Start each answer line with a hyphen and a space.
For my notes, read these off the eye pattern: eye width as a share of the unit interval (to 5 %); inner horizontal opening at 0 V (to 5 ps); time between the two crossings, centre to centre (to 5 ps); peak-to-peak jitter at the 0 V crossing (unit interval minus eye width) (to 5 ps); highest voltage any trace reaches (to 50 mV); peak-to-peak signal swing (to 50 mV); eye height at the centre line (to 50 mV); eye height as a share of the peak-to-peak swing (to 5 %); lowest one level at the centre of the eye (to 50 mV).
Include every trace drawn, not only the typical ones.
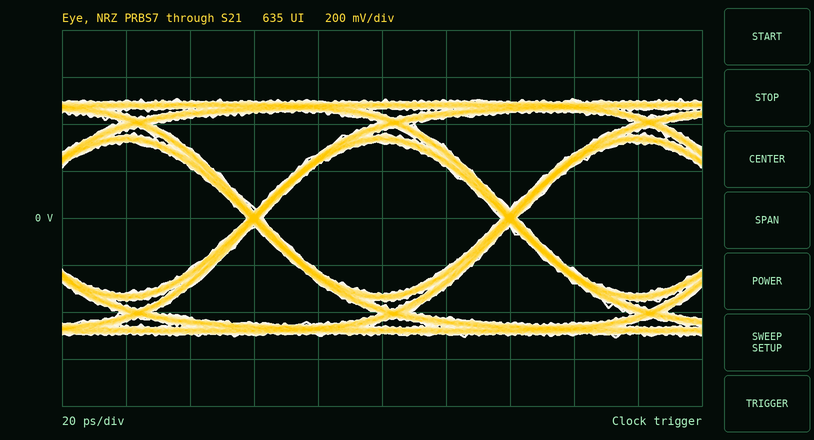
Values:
- 95 %
- 75 ps
- 80 ps
- 5 ps
- 500 mV
- 1.00 V
- 650 mV
- 65 %
- 300 mV
